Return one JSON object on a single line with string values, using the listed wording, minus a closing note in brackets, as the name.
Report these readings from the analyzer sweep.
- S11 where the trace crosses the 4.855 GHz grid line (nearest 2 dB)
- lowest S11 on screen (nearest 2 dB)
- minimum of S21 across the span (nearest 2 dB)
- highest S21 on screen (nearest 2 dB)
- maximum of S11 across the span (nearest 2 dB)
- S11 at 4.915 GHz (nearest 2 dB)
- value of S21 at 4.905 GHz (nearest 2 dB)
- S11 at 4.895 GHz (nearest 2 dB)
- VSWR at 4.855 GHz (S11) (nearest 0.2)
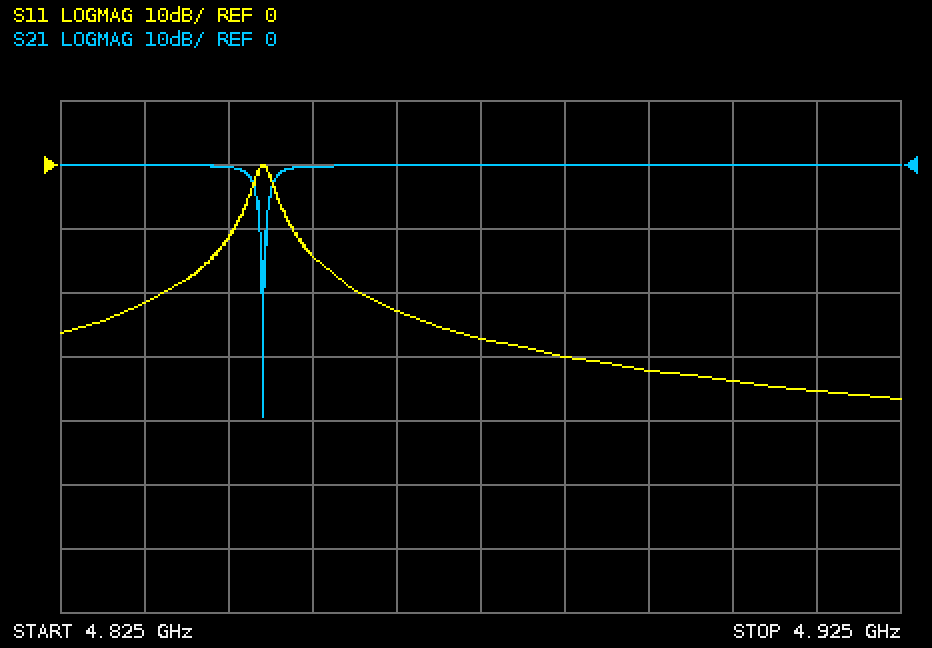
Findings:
{"S11 where the trace crosses the 4.855 GHz grid line": "-14 dB", "lowest S11 on screen": "-36 dB", "minimum of S21 across the span": "-40 dB", "highest S21 on screen": "0 dB", "maximum of S11 across the span": "0 dB", "S11 at 4.915 GHz": "-36 dB", "value of S21 at 4.905 GHz": "0 dB", "S11 at 4.895 GHz": "-32 dB", "VSWR at 4.855 GHz (S11)": "1.4"}
